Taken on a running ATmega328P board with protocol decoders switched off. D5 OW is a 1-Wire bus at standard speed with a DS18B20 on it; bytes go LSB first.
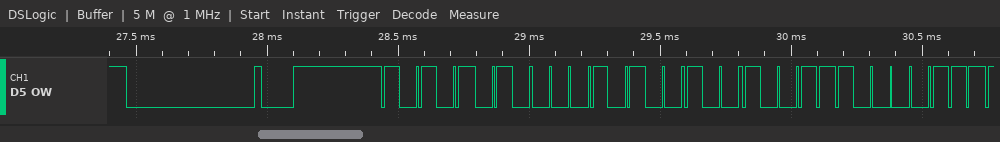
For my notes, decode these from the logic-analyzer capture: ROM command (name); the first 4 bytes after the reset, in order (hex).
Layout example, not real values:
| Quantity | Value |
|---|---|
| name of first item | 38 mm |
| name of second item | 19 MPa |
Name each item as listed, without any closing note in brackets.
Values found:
| Quantity | Value |
|---|---|
| ROM command | Match ROM |
| the first 4 bytes after the reset, in order | 55 28 C9 E1 |
